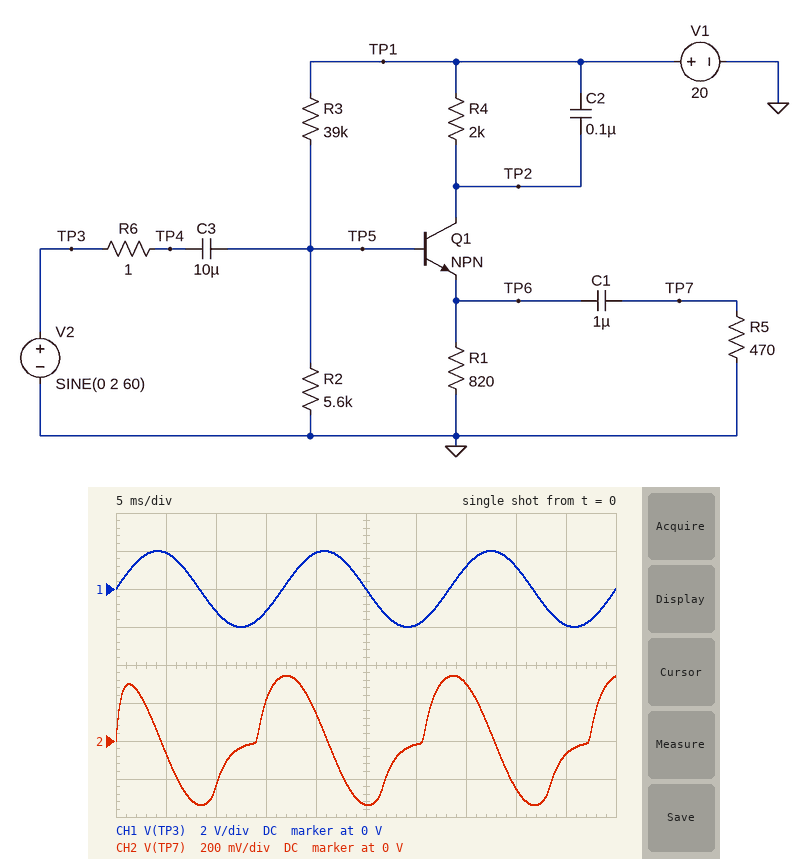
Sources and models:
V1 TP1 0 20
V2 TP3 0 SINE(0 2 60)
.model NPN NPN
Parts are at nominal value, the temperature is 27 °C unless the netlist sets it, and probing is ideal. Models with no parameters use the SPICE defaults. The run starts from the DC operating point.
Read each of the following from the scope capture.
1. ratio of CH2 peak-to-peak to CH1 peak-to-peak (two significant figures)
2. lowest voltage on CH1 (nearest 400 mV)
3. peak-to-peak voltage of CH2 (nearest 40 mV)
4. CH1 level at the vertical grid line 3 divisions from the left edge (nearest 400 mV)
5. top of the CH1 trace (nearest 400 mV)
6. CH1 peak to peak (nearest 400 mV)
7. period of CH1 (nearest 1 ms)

0.17
-2.0 V
680 mV
-1.2 V
2.0 V
4.0 V
17 ms
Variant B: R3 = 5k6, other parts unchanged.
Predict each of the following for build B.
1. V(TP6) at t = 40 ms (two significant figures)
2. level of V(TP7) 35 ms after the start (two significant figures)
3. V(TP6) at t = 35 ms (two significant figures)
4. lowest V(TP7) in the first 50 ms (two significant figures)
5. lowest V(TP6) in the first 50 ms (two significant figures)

6.5 V
210 mV
7.4 V
-290 mV
4.1 V
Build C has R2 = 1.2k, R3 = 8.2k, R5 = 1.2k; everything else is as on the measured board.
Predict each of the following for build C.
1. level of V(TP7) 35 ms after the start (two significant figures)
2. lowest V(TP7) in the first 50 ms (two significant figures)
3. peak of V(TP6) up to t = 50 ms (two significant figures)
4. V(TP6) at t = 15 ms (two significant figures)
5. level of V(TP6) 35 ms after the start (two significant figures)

710 mV
-770 mV
3.6 V
920 mV
3.2 V
